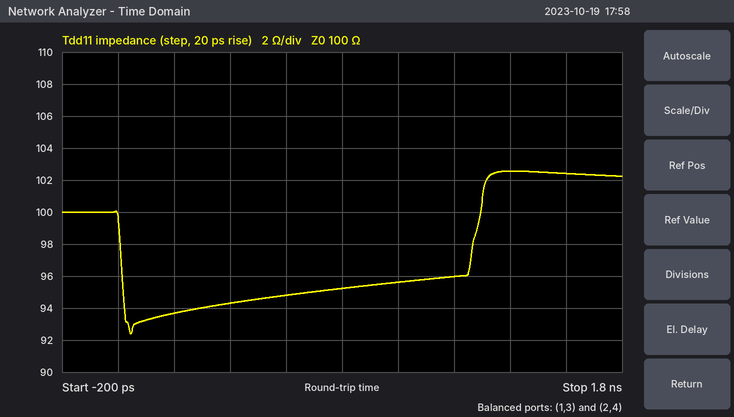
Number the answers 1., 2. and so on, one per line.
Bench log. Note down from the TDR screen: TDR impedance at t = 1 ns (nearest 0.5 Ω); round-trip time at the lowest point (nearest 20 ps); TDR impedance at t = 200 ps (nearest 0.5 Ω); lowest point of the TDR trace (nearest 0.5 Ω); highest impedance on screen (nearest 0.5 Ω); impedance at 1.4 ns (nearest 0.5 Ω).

1. 95.5 Ω
2. 40 ps
3. 93.5 Ω
4. 92.5 Ω
5. 102.5 Ω
6. 102.5 Ω
